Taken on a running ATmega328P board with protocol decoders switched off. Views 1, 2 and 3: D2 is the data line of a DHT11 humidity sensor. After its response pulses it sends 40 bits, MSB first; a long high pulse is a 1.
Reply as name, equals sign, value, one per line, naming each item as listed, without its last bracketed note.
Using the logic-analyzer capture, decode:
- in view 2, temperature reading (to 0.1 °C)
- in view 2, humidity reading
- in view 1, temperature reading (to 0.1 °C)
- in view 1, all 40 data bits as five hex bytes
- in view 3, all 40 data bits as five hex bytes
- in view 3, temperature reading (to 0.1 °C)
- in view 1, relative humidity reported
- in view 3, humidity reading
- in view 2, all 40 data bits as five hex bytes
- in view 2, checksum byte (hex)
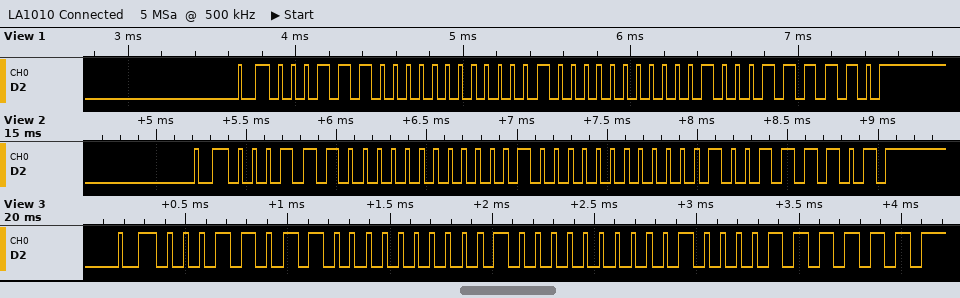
in view 2, temperature reading = 32.1 °C
in view 2, humidity reading = 28 %
in view 1, temperature reading = 32.2 °C
in view 1, all 40 data bits as five hex bytes = 1C 00 20 02 3E
in view 3, all 40 data bits as five hex bytes = 1B 00 20 04 3F
in view 3, temperature reading = 32.4 °C
in view 1, relative humidity reported = 28 %
in view 3, humidity reading = 27 %
in view 2, all 40 data bits as five hex bytes = 1C 00 20 01 3D
in view 2, checksum byte = 0x3D
